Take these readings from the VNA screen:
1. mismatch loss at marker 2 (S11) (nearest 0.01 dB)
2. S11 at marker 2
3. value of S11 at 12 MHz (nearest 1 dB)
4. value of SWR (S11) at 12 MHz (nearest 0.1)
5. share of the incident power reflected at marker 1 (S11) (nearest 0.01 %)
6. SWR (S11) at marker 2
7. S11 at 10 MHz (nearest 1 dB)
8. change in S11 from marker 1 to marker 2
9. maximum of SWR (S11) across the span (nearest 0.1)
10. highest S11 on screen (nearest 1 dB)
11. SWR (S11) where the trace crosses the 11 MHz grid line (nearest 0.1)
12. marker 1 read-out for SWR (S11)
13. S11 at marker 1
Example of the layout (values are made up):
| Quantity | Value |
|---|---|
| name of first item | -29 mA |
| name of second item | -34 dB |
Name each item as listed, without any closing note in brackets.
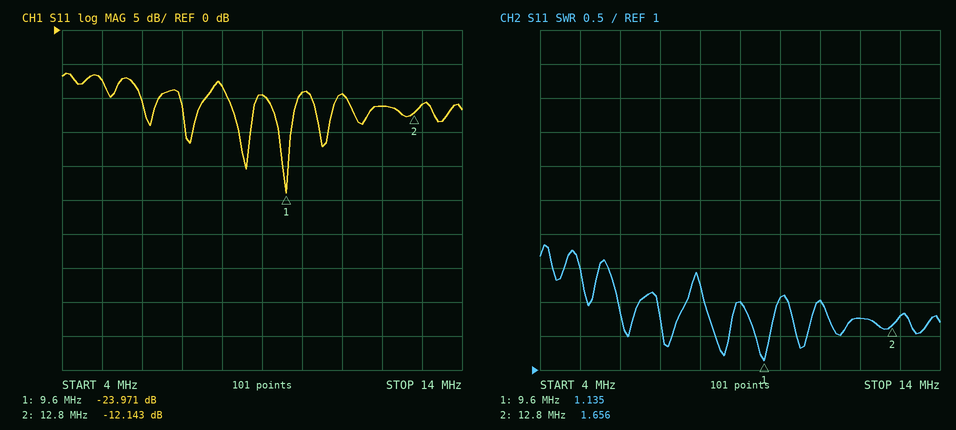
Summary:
| Quantity | Value |
|---|---|
| mismatch loss at marker 2 (S11) | 0.27 dB |
| S11 at marker 2 | -12.143 dB |
| value of S11 at 12 MHz | -11 dB |
| value of SWR (S11) at 12 MHz | 1.8 |
| share of the incident power reflected at marker 1 (S11) | 0.40 % |
| SWR (S11) at marker 2 | 1.656 |
| S11 at 10 MHz | -9 dB |
| change in S11 from marker 1 to marker 2 | 11.828 dB |
| maximum of SWR (S11) across the span | 2.8 |
| highest S11 on screen | -6 dB |
| SWR (S11) where the trace crosses the 11 MHz grid line | 2.0 |
| marker 1 read-out for SWR | 1.135 |
| S11 at marker 1 | -23.971 dB |
